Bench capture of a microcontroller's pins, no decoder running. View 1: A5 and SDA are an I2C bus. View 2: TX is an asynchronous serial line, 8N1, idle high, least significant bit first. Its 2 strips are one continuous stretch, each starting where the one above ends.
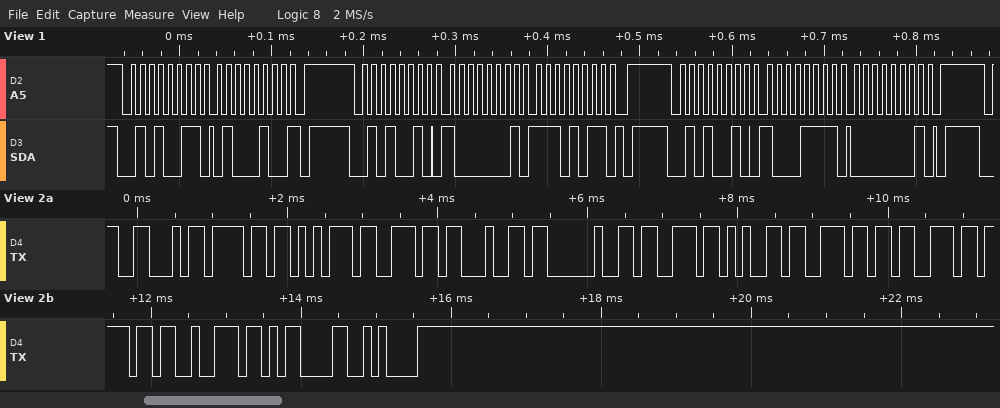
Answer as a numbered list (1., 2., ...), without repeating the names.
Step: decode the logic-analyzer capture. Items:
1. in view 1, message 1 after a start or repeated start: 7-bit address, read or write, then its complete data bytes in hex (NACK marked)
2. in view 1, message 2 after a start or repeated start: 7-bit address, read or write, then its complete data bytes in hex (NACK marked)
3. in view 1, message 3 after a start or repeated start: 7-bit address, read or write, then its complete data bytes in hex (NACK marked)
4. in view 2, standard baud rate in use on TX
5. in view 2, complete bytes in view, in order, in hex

1. 0x29 read: 44 NACK
2. 0x29 write: 81 EB
3. 0x29 write: 8F 01
4. 9600 baud
5. 46 6F 75 6E 64 20 73 65 6E 73 6F 72 0D 0A
